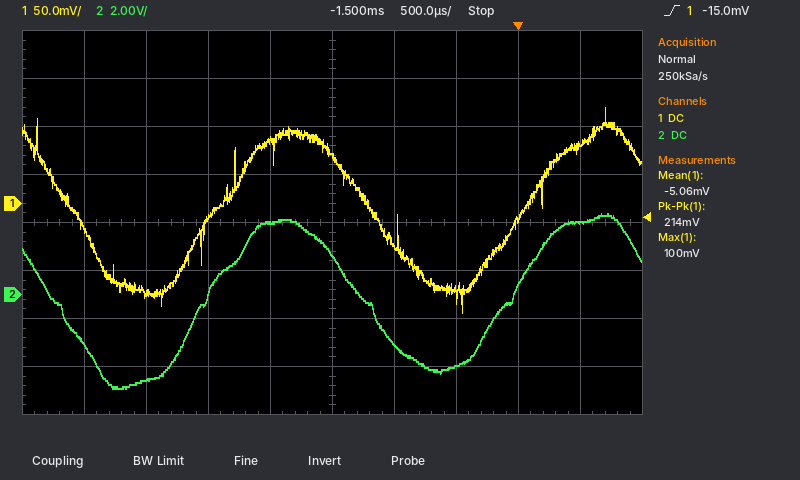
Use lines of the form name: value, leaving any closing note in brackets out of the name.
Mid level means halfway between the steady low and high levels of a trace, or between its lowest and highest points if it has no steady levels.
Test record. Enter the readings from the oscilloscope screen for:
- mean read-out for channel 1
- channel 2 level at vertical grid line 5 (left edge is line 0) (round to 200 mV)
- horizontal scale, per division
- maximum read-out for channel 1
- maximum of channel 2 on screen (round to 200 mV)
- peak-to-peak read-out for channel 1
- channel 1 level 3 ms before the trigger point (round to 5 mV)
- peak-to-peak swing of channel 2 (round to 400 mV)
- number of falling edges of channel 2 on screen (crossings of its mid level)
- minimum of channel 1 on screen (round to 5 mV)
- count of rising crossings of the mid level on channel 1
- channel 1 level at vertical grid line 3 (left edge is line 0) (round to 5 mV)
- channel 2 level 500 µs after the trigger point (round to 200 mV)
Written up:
mean read-out for channel 1: -5.06 mV
channel 2 level at vertical grid line 5 (left edge is line 0): 1.6 V
horizontal scale, per division: 500 µs
maximum read-out for channel 1: 100 mV
maximum of channel 2 on screen: 3.4 V
peak-to-peak read-out for channel 1: 214 mV
channel 1 level 3 ms before the trigger point: -95 mV
peak-to-peak swing of channel 2: 7.2 V
number of falling edges of channel 2 on screen: 2
minimum of channel 1 on screen: -115 mV
count of rising crossings of the mid level on channel 1: 2
channel 1 level at vertical grid line 3 (left edge is line 0): -15 mV
channel 2 level 500 µs after the trigger point: 3.0 V
